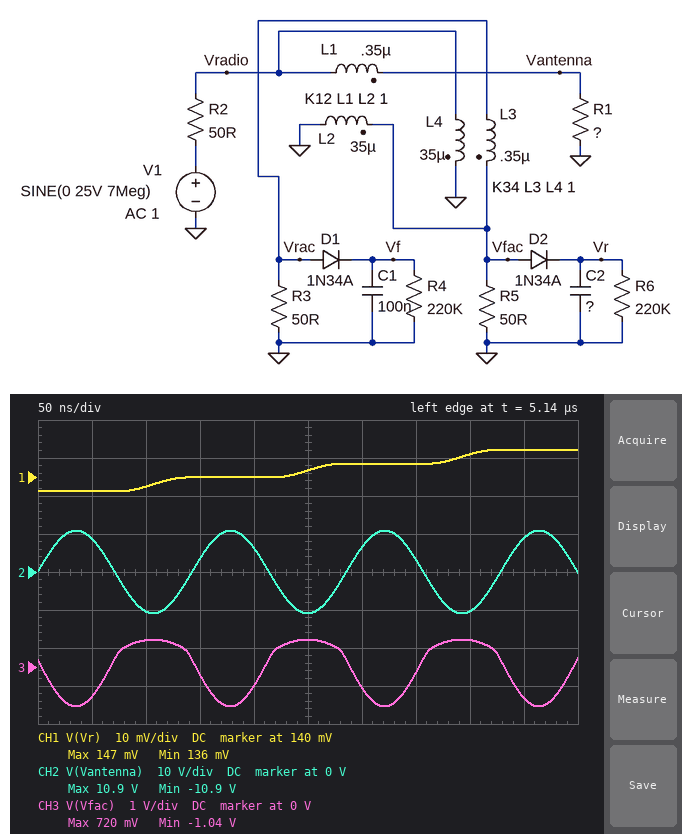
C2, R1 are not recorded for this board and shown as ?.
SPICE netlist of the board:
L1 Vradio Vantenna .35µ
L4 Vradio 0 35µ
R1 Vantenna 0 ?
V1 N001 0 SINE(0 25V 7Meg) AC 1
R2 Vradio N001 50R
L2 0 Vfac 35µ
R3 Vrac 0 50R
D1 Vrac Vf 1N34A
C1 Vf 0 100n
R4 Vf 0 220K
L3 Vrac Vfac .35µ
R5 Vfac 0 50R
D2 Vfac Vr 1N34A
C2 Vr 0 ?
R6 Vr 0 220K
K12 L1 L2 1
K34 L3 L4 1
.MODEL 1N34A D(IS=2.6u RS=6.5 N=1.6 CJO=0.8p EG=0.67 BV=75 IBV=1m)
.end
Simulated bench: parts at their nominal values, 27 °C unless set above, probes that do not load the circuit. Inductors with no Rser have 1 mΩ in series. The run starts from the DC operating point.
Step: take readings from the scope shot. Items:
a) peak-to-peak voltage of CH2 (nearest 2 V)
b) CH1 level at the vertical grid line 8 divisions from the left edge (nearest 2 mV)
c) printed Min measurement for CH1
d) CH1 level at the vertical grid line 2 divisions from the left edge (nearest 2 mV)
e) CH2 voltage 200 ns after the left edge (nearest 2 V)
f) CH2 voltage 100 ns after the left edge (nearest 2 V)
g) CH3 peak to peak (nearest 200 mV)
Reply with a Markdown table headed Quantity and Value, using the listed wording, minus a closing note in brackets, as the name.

| Quantity | Value |
|---|---|
| peak-to-peak voltage of CH2 | 22 V |
| CH1 level at the vertical grid line 8 divisions from the left edge | 146 mV |
| printed Min measurement for CH1 | 136 mV |
| CH1 level at the vertical grid line 2 divisions from the left edge | 138 mV |
| CH2 voltage 200 ns after the left edge | 6 V |
| CH2 voltage 100 ns after the left edge | -10 V |
| CH3 peak to peak | 1.8 V |
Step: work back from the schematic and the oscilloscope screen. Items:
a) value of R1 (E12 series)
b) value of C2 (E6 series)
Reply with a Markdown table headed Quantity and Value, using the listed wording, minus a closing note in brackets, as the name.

| Quantity | Value |
|---|---|
| value of R1 | 39 Ω |
| value of C2 | 330 nF |
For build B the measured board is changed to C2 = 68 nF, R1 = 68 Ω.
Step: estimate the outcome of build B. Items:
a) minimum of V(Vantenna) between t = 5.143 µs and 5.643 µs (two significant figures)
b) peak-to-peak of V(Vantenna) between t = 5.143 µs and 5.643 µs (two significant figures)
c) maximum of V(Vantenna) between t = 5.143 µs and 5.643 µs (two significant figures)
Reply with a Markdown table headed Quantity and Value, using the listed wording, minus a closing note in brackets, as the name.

| Quantity | Value |
|---|---|
| minimum of V(Vantenna) between t = 5.143 µs and 5.643 µs | -14 V |
| peak-to-peak of V(Vantenna) between t = 5.143 µs and 5.643 µs | 29 V |
| maximum of V(Vantenna) between t = 5.143 µs and 5.643 µs | 14 V |
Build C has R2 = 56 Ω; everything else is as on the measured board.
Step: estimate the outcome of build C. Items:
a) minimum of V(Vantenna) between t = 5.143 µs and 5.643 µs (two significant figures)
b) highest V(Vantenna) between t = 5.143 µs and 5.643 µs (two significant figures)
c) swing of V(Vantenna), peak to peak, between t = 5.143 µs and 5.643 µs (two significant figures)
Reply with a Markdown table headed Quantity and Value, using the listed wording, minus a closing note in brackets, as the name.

| Quantity | Value |
|---|---|
| minimum of V(Vantenna) between t = 5.143 µs and 5.643 µs | -10 V |
| highest V(Vantenna) between t = 5.143 µs and 5.643 µs | 10 V |
| swing of V(Vantenna), peak to peak, between t = 5.143 µs and 5.643 µs | 20 V |
